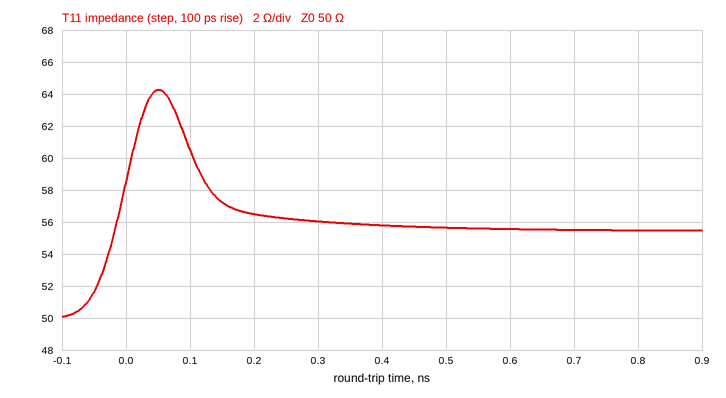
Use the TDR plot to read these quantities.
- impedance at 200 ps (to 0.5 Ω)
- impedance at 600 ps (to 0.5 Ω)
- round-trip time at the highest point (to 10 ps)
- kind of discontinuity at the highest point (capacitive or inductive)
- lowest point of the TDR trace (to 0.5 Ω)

56.5 Ω
55.5 Ω
50 ps
inductive
50.0 Ω
